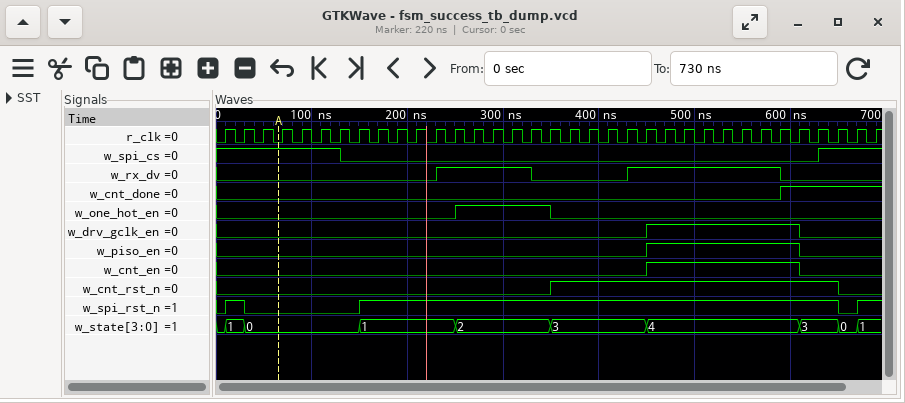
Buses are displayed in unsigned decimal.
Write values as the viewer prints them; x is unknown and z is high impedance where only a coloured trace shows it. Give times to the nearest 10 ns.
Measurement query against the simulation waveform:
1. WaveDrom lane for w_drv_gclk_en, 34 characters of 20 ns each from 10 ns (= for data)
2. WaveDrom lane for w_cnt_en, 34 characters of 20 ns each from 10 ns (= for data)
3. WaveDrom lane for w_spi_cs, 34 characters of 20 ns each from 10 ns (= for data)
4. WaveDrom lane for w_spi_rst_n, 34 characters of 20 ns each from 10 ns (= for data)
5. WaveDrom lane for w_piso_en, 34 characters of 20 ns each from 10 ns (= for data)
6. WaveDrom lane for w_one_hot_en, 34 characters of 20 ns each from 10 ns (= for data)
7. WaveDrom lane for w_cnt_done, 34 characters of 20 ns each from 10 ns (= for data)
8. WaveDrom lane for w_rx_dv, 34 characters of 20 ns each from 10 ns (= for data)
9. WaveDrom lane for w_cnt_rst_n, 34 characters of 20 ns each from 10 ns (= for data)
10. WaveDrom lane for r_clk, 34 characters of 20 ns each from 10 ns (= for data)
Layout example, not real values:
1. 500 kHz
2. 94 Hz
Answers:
1. {name: 'w_drv_gclk_en', wave: '0.....................1.......0...'}
2. {name: 'w_cnt_en', wave: '0.....................1.......0...'}
3. {name: 'w_spi_cs', wave: '1.....0........................1..'}
4. {name: 'w_spi_rst_n', wave: '10.....1........................01'}
5. {name: 'w_piso_en', wave: '0.....................1.......0...'}
6. {name: 'w_one_hot_en', wave: '0...........1....0................'}
7. {name: 'w_cnt_done', wave: '0............................1....'}
8. {name: 'w_rx_dv', wave: '0..........1....0....1.......0....'}
9. {name: 'w_cnt_rst_n', wave: '0................1..............0.'}
10. {name: 'r_clk', wave: 'p.................................'}
